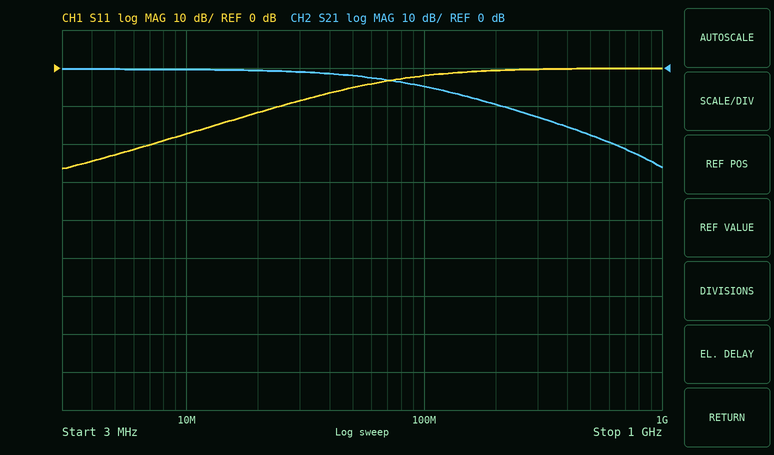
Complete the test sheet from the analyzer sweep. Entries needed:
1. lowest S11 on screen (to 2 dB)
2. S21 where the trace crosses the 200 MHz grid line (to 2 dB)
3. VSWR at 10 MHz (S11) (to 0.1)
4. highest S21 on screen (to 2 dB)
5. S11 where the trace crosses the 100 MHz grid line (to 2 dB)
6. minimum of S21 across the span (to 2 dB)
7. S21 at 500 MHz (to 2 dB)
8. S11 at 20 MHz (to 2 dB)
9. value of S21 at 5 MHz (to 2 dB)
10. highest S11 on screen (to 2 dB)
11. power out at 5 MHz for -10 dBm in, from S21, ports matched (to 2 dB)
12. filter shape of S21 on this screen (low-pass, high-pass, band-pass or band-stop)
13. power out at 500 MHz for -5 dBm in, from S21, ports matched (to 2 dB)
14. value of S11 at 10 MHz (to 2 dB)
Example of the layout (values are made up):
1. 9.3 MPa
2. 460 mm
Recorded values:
1. -26 dB
2. -10 dB
3. 1.3
4. 0 dB
5. -2 dB
6. -26 dB
7. -18 dB
8. -12 dB
9. 0 dB
10. 0 dB
11. -10 dBm
12. low-pass
13. -22 dBm
14. -18 dB
